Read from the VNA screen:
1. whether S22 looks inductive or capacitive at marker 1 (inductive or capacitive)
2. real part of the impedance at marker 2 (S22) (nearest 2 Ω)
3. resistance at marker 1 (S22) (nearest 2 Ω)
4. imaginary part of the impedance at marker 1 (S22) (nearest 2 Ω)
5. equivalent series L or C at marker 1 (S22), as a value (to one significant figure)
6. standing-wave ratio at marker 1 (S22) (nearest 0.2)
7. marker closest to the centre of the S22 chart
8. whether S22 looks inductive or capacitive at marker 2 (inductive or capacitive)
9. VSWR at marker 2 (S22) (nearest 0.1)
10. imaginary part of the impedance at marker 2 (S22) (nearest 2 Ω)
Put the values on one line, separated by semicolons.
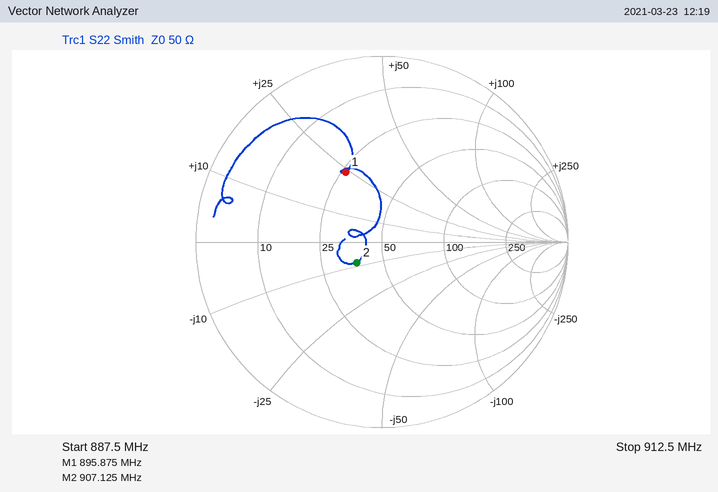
inductive; 38 Ω; 26 Ω; +24 Ω; 4 nH; 2.4; marker 2; capacitive; 1.4; -8 Ω
